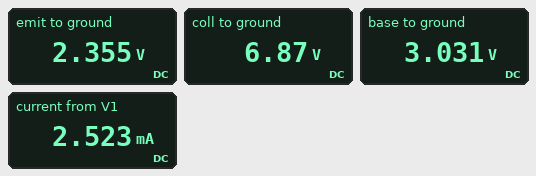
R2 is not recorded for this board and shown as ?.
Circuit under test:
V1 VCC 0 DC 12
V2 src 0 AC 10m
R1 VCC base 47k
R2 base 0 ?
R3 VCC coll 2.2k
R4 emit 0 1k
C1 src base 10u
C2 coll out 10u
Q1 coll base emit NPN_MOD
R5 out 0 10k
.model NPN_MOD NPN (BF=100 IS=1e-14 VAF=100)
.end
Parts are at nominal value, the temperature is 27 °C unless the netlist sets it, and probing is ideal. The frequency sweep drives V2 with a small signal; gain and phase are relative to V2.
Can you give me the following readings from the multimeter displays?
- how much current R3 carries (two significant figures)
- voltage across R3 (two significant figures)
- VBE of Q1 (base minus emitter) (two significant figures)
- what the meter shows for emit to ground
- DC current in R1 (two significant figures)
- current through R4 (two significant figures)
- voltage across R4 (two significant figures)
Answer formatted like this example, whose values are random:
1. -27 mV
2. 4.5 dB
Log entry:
1. 2.3 mA
2. 5.1 V
3. 680 mV
4. 2.355 V
5. 190 µA
6. 2.4 mA
7. 2.4 V
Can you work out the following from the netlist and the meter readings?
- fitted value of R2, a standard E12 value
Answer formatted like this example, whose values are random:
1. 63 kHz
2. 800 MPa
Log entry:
1. 18 kΩ
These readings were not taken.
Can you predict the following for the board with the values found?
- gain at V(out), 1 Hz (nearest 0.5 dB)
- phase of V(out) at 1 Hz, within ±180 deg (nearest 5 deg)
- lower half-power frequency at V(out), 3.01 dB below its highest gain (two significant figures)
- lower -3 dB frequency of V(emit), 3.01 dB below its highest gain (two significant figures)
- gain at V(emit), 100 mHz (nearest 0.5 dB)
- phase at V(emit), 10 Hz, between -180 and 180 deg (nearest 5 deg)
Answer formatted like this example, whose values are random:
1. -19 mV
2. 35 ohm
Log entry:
1. -4.0 dB
2. -75 deg
3. 2.1 Hz
4. 1.4 Hz
5. -23.0 dB
6. 10 deg
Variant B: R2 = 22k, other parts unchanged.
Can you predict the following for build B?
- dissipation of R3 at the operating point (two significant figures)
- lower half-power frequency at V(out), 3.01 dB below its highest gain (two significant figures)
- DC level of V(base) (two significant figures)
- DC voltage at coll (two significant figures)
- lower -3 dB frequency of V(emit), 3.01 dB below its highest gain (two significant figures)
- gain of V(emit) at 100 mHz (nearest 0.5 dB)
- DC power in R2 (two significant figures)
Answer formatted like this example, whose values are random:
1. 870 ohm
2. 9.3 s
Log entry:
1. 16 mW
2. 2.0 Hz
3. 3.4 V
4. 6.0 V
5. 1.2 Hz
6. -22.0 dB
7. 530 µW
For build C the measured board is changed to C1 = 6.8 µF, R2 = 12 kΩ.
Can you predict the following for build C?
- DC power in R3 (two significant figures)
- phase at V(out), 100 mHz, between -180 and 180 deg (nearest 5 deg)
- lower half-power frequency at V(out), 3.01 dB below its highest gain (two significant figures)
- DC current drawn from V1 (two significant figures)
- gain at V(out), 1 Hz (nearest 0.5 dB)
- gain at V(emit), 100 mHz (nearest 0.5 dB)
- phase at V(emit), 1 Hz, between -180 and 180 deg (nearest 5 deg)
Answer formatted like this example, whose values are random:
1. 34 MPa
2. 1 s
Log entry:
1. 5.7 mW
2. -5 deg
3. 3.2 Hz
4. 1.8 mA
5. -8.5 dB
6. -28.5 dB
7. 70 deg
